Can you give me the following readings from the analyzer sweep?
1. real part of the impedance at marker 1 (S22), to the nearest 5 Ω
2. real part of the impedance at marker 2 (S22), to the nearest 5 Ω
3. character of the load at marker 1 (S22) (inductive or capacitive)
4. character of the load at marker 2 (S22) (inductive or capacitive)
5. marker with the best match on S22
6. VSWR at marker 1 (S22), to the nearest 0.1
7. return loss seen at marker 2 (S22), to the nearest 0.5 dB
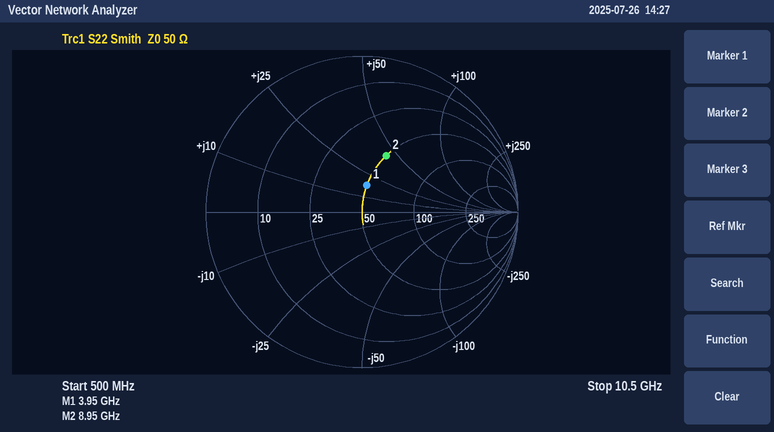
50 Ω
50 Ω
inductive
inductive
marker 1
1.4
8.0 dB
